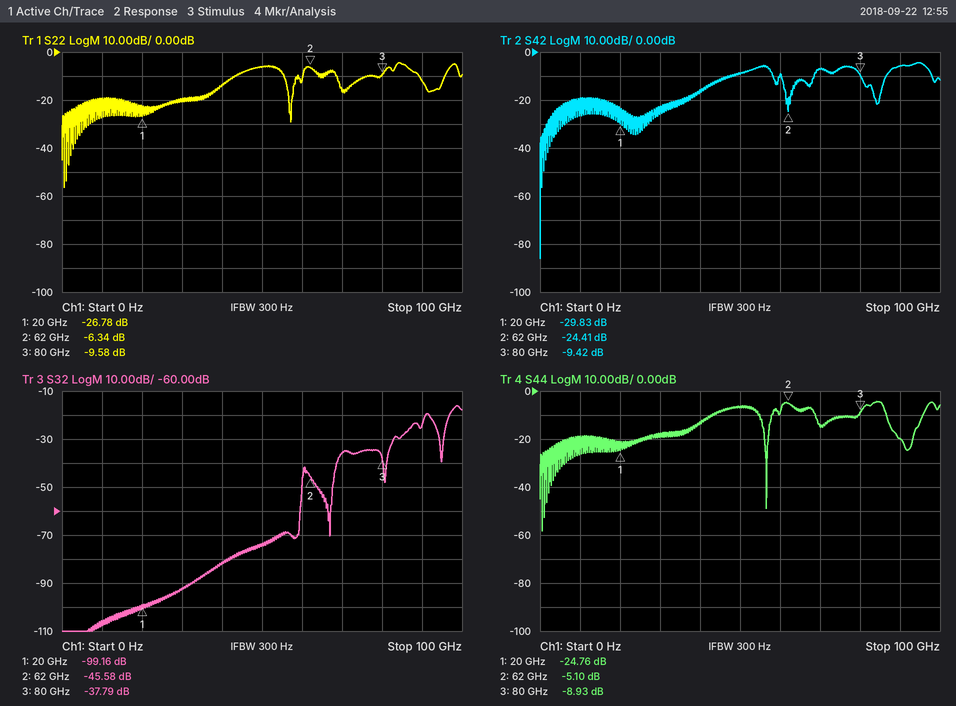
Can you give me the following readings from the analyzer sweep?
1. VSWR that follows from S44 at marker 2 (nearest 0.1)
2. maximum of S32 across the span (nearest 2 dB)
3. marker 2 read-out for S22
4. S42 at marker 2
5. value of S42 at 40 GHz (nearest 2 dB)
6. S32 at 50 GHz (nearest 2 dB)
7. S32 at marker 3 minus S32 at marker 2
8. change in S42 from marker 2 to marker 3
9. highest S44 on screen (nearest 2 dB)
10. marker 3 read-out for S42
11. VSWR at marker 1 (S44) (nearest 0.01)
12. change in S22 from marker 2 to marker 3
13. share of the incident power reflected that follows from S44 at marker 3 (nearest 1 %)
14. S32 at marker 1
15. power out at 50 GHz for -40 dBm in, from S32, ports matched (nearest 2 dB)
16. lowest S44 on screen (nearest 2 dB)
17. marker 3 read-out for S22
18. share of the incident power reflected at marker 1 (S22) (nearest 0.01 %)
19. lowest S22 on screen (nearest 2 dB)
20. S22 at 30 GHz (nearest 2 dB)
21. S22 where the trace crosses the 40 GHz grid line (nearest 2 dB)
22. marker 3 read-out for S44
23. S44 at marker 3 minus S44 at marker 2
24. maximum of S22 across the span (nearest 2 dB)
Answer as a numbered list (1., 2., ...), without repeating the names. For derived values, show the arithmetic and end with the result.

1. (1 + 0.5559)/(1 − 0.5559) ≈ 3.5
2. -16 dB
3. -6.34 dB
4. -24.41 dB
5. -16 dB
6. -74 dB
7. -37.79 − (-45.58) = 7.79 dB
8. -9.42 − (-24.41) = 14.99 dB
9. -4 dB
10. -9.42 dB
11. (1 + 0.0578)/(1 − 0.0578) ≈ 1.12
12. -9.58 − (-6.34) = -3.24 dB
13. 10^(-8.93/10) ≈ 13 %
14. -99.16 dB
15. -40 dBm + (-74 dB) = -114 dBm
16. -58 dB
17. -9.58 dB
18. 10^(-26.78/10) ≈ 0.21 %
19. -56 dB
20. -20 dB
21. -14 dB
22. -8.93 dB
23. -8.93 − (-5.1) = -3.83 dB
24. -4 dB
